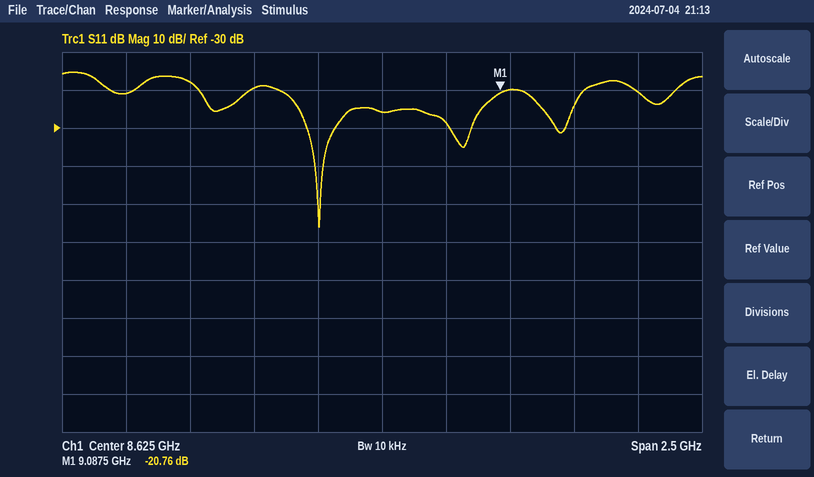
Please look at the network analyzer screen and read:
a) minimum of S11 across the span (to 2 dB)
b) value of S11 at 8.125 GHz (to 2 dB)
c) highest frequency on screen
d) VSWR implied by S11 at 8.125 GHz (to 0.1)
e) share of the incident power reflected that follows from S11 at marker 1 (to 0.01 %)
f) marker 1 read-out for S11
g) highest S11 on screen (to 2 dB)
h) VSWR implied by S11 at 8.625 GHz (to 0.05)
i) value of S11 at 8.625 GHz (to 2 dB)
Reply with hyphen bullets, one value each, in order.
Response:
- -56 dB
- -20 dB
- 9.875 GHz
- 1.2
- 0.84 %
- -20.76 dB
- -16 dB
- 1.10
- -26 dB
